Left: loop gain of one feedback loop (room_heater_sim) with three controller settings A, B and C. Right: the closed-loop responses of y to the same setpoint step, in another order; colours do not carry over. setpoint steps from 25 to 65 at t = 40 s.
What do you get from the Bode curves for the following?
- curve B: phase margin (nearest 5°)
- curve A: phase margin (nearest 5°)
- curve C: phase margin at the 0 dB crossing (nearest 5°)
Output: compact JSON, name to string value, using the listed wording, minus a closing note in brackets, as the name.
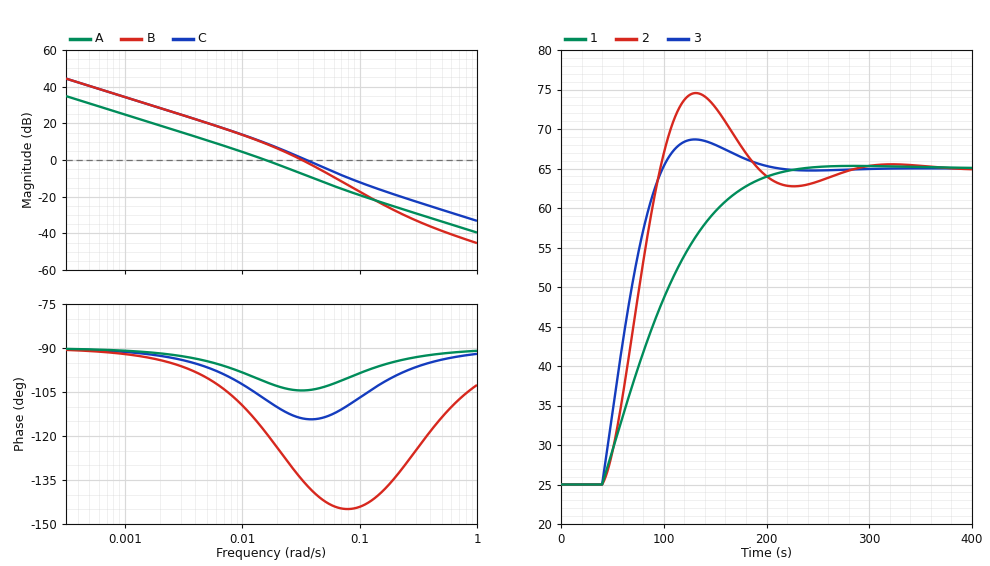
{"curve B: phase margin": "45°", "curve A: phase margin": "80°", "curve C: phase margin at the 0 dB crossing": "65°"}
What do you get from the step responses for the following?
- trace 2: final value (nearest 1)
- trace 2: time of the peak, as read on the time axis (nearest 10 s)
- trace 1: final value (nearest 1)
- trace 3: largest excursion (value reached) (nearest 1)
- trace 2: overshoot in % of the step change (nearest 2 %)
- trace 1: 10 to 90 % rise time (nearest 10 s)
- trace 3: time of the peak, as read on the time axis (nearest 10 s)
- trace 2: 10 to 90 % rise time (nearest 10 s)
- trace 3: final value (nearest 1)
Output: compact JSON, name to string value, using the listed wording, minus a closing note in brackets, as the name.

{"trace 2: final value": "65", "trace 2: time of the peak, as read on the time axis": "130 s", "trace 1: final value": "65", "trace 3: largest excursion (value reached)": "69", "trace 2: overshoot in % of the step change": "24 %", "trace 1: 10 to 90 % rise time": "110 s", "trace 3: time of the peak, as read on the time axis": "130 s", "trace 2: 10 to 90 % rise time": "40 s", "trace 3: final value": "65"}
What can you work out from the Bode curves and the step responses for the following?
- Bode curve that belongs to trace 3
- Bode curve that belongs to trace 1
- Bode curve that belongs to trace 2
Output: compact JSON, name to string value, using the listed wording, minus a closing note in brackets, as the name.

{"Bode curve that belongs to trace 3": "C", "Bode curve that belongs to trace 1": "A", "Bode curve that belongs to trace 2": "B"}
